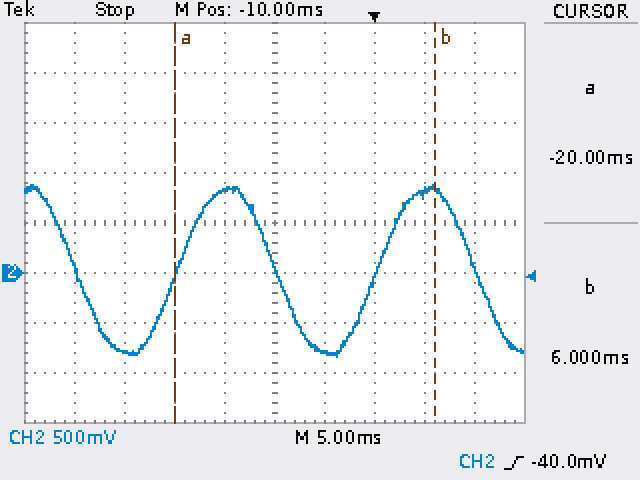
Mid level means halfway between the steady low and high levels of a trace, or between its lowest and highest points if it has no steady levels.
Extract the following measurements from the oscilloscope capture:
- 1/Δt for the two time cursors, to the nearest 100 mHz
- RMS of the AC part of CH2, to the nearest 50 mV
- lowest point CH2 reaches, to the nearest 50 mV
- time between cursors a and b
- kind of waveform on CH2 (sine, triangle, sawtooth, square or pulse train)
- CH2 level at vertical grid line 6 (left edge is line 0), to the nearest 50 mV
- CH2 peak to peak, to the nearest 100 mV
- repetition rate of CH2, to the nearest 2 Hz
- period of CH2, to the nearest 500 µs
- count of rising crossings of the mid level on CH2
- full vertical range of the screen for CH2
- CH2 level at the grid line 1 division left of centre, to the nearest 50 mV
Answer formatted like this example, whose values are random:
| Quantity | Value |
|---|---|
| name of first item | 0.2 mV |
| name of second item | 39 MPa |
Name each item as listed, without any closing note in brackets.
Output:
| Quantity | Value |
|---|---|
| 1/Δt for the two time cursors, to the nearest 100 mHz | 38.5 Hz |
| RMS of the AC part of CH2, to the nearest 50 mV | 600 mV |
| lowest point CH2 reaches, to the nearest 50 mV | -850 mV |
| time between cursors a and b | 26.0 ms |
| kind of waveform on CH2 | sine |
| CH2 level at vertical grid line 6 (left edge is line 0), to the nearest 50 mV | -800 mV |
| CH2 peak to peak, to the nearest 100 mV | 1.70 V |
| repetition rate of CH2, to the nearest 2 Hz | 50 Hz |
| period of CH2, to the nearest 500 µs | 20.0 ms |
| count of rising crossings of the mid level on CH2 | 2 |
| full vertical range of the screen for CH2 | 4 V |
| CH2 level at the grid line 1 division left of centre, to the nearest 50 mV | 850 mV |
